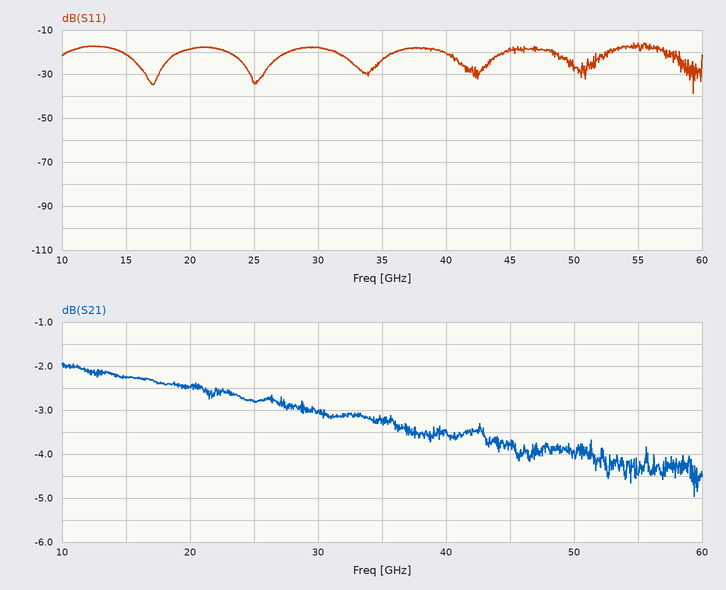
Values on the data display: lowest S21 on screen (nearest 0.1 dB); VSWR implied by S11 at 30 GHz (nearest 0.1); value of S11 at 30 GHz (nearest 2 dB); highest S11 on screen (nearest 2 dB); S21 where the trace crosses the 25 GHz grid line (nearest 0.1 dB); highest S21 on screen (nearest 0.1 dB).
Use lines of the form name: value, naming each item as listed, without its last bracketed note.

lowest S21 on screen: -5.0 dB
VSWR implied by S11 at 30 GHz: 1.3
value of S11 at 30 GHz: -18 dB
highest S11 on screen: -16 dB
S21 where the trace crosses the 25 GHz grid line: -2.8 dB
highest S21 on screen: -1.9 dB
